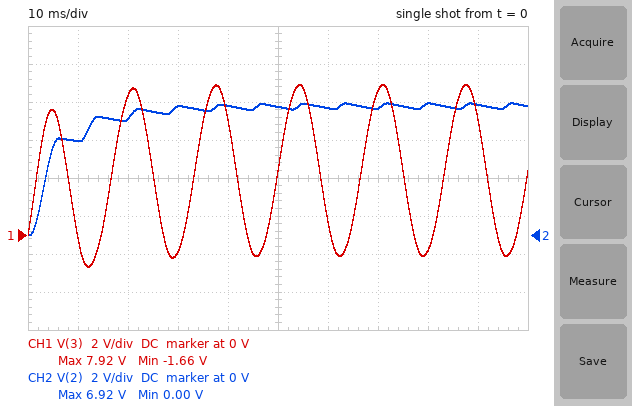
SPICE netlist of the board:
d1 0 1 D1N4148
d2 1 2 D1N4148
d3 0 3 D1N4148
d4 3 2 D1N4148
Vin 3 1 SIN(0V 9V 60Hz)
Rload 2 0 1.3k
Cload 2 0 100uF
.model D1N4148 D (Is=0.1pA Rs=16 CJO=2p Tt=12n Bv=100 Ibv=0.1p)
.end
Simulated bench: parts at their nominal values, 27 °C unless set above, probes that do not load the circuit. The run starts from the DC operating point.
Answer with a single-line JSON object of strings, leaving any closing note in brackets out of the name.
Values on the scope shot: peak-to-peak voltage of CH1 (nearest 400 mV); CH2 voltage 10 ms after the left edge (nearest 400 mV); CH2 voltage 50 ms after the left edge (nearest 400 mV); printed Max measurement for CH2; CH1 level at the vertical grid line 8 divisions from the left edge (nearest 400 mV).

{"peak-to-peak voltage of CH1": "9.6 V", "CH2 voltage 10 ms after the left edge": "4.8 V", "CH2 voltage 50 ms after the left edge": "6.8 V", "printed Max measurement for CH2": "6.92 V", "CH1 level at the vertical grid line 8 divisions from the left edge": "-800 mV"}
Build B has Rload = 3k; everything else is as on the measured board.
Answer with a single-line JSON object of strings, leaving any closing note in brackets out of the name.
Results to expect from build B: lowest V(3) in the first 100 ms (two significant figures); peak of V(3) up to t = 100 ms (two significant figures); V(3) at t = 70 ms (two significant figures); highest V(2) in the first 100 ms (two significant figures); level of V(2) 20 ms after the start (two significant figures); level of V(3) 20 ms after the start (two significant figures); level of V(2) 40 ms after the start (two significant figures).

{"lowest V(3) in the first 100 ms": "-1.6 V", "peak of V(3) up to t = 100 ms": "8.1 V", "V(3) at t = 70 ms": "7.8 V", "highest V(2) in the first 100 ms": "7.2 V", "level of V(2) 20 ms after the start": "6.3 V", "level of V(3) 20 ms after the start": "7.4 V", "level of V(2) 40 ms after the start": "7.1 V"}
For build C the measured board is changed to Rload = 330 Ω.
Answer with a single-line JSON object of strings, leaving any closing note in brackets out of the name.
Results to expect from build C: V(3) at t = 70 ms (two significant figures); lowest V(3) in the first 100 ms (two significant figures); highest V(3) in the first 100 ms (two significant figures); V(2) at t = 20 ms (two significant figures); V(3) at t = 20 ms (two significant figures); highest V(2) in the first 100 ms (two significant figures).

{"V(3) at t = 70 ms": "7.0 V", "lowest V(3) in the first 100 ms": "-1.9 V", "highest V(3) in the first 100 ms": "7.4 V", "V(2) at t = 20 ms": "5.3 V", "V(3) at t = 20 ms": "6.9 V", "highest V(2) in the first 100 ms": "6.1 V"}
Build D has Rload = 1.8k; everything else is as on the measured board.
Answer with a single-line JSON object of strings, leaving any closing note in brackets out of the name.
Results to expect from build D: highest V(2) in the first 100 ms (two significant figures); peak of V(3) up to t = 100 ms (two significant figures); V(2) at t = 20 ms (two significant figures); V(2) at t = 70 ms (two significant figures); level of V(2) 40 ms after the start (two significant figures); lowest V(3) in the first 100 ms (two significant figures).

{"highest V(2) in the first 100 ms": "7.1 V", "peak of V(3) up to t = 100 ms": "8.0 V", "V(2) at t = 20 ms": "6.2 V", "V(2) at t = 70 ms": "6.8 V", "level of V(2) 40 ms after the start": "6.9 V", "lowest V(3) in the first 100 ms": "-1.6 V"}
